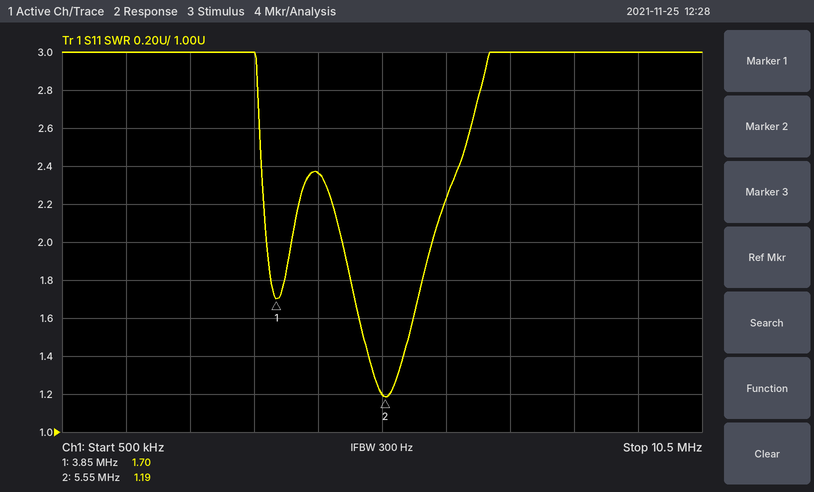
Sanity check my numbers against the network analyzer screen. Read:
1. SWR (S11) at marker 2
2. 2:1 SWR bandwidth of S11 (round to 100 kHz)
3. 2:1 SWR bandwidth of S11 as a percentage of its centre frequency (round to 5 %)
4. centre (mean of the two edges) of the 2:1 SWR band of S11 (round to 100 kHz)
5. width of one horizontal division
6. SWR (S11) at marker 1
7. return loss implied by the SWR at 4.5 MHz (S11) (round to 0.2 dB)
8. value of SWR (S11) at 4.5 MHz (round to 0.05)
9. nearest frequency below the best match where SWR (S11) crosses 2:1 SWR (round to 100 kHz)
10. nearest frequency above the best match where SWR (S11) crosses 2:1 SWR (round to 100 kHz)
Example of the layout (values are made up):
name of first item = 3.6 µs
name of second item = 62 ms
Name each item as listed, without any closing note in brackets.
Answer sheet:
SWR (S11) at marker 2 = 1.19
2:1 SWR bandwidth of S11 = 1.4 MHz
2:1 SWR bandwidth of S11 as a percentage of its centre frequency = 25 %
centre (mean of the two edges) of the 2:1 SWR band of S11 = 5.6 MHz
width of one horizontal division = 1 MHz
SWR (S11) at marker 1 = 1.70
return loss implied by the SWR at 4.5 MHz (S11) = 7.8 dB
value of SWR (S11) at 4.5 MHz = 2.35
nearest frequency below the best match where SWR (S11) crosses 2:1 SWR = 4.9 MHz
nearest frequency above the best match where SWR (S11) crosses 2:1 SWR = 6.3 MHz
